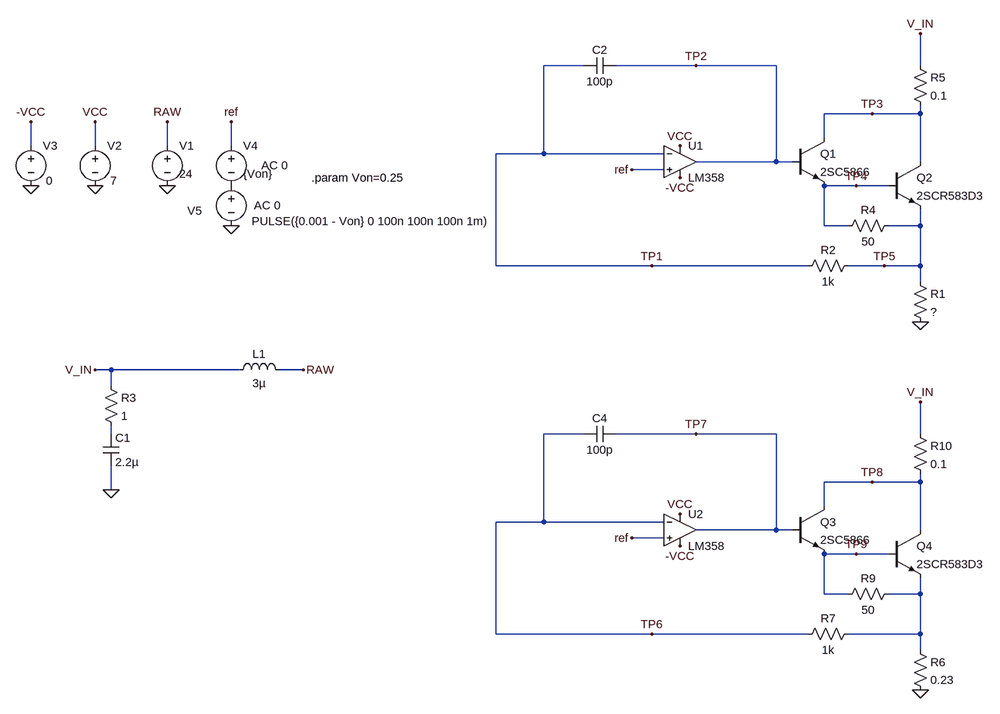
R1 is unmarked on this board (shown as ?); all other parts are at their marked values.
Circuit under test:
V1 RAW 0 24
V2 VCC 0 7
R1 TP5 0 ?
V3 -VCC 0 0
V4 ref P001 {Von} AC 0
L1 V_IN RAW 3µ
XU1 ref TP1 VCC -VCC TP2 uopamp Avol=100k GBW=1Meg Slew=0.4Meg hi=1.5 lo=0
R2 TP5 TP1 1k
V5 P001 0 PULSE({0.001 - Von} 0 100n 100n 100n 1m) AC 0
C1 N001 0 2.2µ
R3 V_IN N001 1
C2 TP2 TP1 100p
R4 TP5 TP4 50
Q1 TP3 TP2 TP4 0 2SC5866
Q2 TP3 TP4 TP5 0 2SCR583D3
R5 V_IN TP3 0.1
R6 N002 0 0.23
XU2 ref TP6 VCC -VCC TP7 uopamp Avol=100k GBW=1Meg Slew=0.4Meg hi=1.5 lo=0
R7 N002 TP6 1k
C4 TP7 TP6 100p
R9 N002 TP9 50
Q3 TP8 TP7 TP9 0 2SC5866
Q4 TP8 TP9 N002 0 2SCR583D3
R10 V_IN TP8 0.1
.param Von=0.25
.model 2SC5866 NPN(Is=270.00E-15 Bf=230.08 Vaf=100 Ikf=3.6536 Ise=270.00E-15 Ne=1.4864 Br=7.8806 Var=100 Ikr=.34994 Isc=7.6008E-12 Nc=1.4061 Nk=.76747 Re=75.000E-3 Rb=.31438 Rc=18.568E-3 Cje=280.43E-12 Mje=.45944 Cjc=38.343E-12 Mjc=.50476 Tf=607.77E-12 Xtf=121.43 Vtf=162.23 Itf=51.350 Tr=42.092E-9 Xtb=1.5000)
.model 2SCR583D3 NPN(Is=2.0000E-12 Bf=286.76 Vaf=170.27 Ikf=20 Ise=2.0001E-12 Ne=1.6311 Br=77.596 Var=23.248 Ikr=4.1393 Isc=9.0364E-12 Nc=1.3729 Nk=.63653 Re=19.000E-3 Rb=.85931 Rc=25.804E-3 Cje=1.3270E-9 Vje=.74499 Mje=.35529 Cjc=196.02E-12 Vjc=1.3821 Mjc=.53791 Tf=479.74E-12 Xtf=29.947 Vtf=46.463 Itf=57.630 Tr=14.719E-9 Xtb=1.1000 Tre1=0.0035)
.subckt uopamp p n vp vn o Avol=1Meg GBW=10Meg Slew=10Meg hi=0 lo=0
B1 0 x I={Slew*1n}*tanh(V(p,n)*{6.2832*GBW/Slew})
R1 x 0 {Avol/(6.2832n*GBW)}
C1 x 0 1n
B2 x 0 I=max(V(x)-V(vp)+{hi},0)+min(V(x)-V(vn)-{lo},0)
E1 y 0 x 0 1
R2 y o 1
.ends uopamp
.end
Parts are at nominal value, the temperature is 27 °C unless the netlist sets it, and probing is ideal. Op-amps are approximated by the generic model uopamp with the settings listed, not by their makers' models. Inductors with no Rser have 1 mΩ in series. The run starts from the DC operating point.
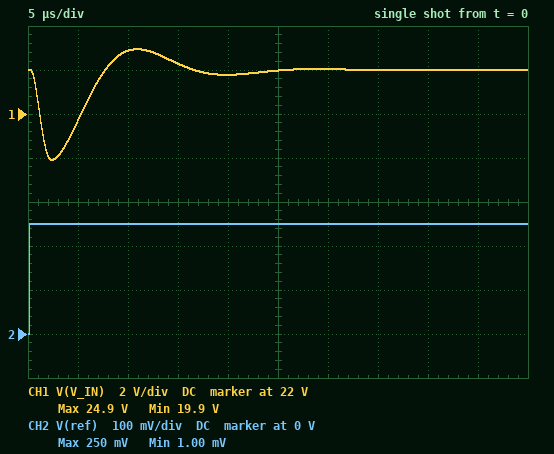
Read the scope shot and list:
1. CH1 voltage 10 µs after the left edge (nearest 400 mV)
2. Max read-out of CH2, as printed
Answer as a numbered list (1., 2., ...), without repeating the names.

1. 24.8 V
2. 250 mV
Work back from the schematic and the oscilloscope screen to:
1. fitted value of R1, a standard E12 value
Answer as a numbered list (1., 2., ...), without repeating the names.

1. 0.082 Ω
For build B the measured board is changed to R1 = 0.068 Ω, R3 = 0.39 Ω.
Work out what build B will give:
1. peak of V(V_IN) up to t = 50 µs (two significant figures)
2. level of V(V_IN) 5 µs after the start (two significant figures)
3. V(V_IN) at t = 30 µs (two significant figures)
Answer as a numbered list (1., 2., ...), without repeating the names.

1. 27 V
2. 20 V
3. 25 V
